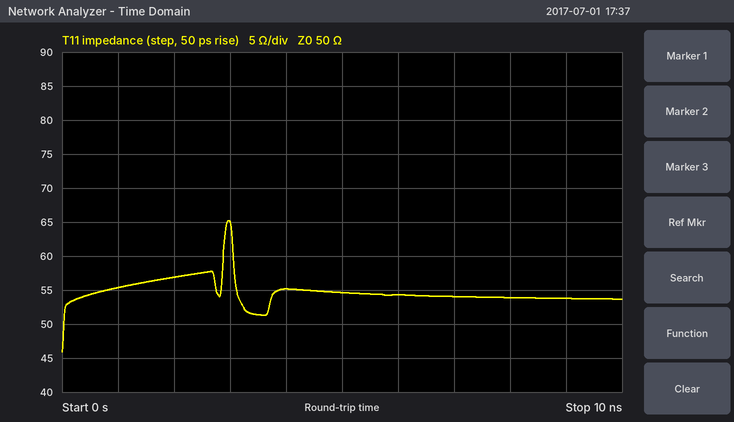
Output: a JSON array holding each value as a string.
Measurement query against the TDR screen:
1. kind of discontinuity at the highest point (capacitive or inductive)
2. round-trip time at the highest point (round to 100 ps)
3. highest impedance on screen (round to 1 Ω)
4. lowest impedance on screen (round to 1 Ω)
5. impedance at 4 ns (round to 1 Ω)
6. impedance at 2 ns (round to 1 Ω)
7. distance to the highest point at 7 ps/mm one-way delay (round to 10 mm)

["inductive", "3.0 ns", "65 Ω", "46 Ω", "55 Ω", "57 Ω", "210 mm"]
